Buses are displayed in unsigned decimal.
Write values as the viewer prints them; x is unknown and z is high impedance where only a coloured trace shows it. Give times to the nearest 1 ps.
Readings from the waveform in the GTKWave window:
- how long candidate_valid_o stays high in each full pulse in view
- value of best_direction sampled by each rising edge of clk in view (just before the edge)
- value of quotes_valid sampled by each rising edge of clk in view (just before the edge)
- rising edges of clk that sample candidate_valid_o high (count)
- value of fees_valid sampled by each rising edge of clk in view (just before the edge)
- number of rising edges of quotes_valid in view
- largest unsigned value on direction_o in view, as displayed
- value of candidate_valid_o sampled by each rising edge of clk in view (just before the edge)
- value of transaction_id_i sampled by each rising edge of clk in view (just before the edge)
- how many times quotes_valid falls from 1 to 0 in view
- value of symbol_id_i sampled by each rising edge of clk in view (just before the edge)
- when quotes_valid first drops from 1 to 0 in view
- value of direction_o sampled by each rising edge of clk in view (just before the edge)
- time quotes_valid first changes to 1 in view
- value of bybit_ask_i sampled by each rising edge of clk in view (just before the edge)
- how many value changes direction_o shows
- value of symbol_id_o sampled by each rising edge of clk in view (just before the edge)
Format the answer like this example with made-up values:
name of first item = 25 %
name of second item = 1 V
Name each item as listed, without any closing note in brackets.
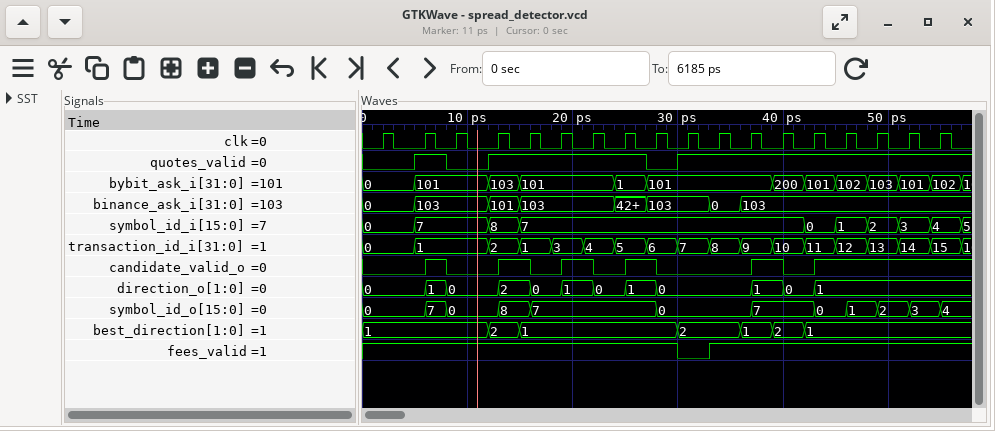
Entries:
how long candidate_valid_o stays high in each full pulse in view = 2 ps, 3 ps, 3 ps, 3 ps, 3 ps
value of best_direction sampled by each rising edge of clk in view = 1, 1, 1, 2, 1, 1, 1, 1, 1, 2, 2, 1, 2, 1, 1, 1, 1, 1
value of quotes_valid sampled by each rising edge of clk in view = 0 1 0 1 1 1 1 1 0 1 1 1 1 1 1 1 1 1
rising edges of clk that sample candidate_valid_o high = 8
value of fees_valid sampled by each rising edge of clk in view = 1 1 1 1 1 1 1 1 1 0 1 1 1 1 1 1 1 1
number of rising edges of quotes_valid in view = 3
largest unsigned value on direction_o in view, as displayed = 2
value of candidate_valid_o sampled by each rising edge of clk in view = 0 0 0 0 1 0 1 0 1 0 0 0 1 0 1 1 1 1
value of transaction_id_i sampled by each rising edge of clk in view = 0, 1, 1, 2, 1, 3, 4, 5, 6, 7, 8, 9, 10, 11, 12, 13, 14, 15
how many times quotes_valid falls from 1 to 0 in view = 2
value of symbol_id_i sampled by each rising edge of clk in view = 0, 7, 7, 8, 7, 7, 7, 7, 7, 7, 7, 7, 7, 0, 1, 2, 3, 4
when quotes_valid first drops from 1 to 0 in view = 8 ps
value of direction_o sampled by each rising edge of clk in view = 0, 0, 0, 0, 2, 0, 1, 0, 1, 0, 0, 0, 1, 0, 1, 1, 1, 1
time quotes_valid first changes to 1 in view = 5 ps
value of bybit_ask_i sampled by each rising edge of clk in view = 0, 101, 101, 103, 101, 101, 101, 1, 101, 101, 101, 101, 200, 101, 102, 103, 101, 102
how many value changes direction_o shows = 11
value of symbol_id_o sampled by each rising edge of clk in view = 0, 0, 0, 0, 8, 7, 7, 7, 7, 0, 0, 0, 7, 7, 0, 1, 2, 3
